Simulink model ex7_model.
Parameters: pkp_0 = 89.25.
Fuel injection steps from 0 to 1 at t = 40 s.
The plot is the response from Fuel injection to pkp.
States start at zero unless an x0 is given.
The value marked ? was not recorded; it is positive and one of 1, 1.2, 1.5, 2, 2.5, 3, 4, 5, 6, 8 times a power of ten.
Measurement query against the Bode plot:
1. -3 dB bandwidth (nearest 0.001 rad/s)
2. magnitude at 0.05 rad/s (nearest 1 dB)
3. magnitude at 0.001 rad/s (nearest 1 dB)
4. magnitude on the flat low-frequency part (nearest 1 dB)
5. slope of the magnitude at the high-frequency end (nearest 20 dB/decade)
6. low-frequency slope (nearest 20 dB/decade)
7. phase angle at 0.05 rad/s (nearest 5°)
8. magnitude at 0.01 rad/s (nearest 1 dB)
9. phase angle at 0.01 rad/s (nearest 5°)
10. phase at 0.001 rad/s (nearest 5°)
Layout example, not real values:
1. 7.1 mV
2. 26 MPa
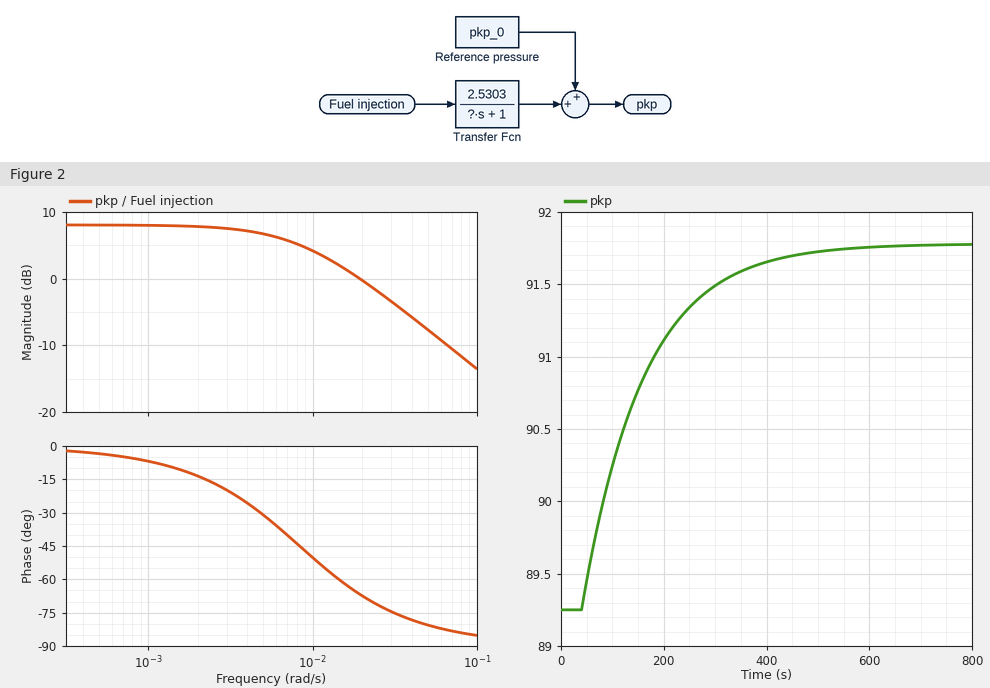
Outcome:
1. 0.008 rad/s
2. -8 dB
3. 8 dB
4. 8 dB
5. -20 dB/decade
6. 0 dB/decade
7. -80°
8. 4 dB
9. -50°
10. -5°
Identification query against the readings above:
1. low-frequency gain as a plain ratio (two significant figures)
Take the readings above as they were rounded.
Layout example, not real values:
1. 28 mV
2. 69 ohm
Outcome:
1. 2.5
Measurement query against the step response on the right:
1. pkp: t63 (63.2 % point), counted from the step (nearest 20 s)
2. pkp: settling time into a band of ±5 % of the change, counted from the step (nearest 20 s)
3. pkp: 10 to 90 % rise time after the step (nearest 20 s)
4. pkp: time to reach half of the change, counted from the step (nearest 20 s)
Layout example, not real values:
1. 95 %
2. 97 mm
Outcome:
1. 120 s
2. 360 s
3. 260 s
4. 80 s
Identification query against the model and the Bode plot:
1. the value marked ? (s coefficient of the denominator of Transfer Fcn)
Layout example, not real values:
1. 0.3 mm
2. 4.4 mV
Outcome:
1. 120
